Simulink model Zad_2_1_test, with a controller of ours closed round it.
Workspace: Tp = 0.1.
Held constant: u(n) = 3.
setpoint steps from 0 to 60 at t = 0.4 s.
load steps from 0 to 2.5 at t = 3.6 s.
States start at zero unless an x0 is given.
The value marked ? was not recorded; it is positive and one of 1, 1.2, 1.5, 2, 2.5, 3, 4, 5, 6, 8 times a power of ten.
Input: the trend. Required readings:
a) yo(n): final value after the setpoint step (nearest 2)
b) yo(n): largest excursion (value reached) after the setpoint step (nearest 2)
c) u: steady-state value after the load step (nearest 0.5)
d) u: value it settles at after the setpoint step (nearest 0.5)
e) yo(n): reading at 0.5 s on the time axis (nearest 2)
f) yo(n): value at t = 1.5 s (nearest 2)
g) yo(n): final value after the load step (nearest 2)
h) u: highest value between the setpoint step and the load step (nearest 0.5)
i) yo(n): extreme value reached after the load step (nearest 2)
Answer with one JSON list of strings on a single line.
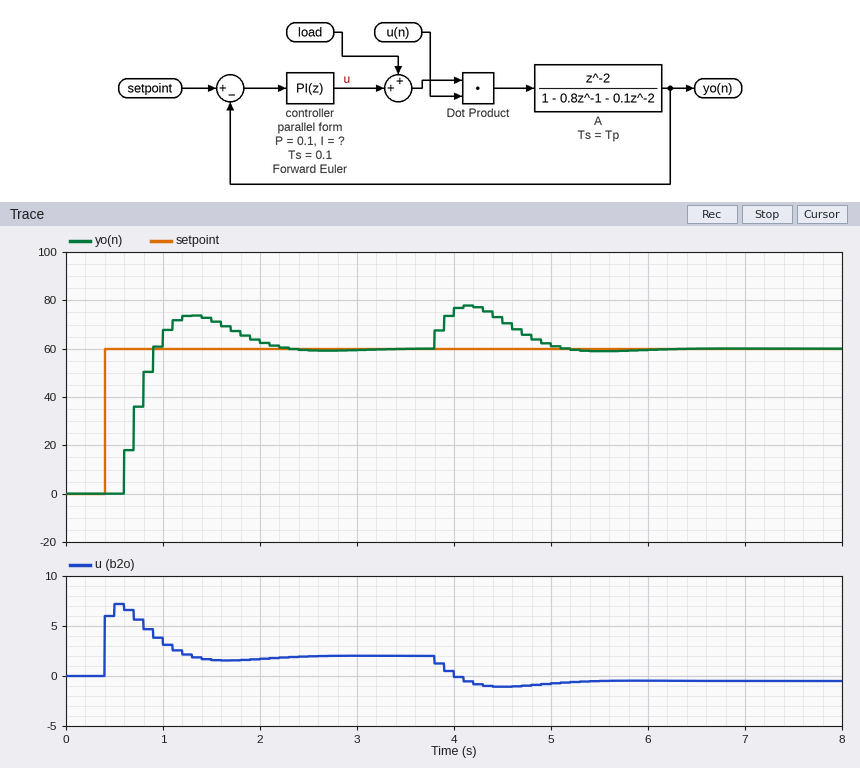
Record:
["60", "74", "-0.5", "2.0", "0", "72", "60", "7.0", "78"]
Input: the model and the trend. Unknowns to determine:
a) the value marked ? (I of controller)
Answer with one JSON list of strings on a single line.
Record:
["0.2"]
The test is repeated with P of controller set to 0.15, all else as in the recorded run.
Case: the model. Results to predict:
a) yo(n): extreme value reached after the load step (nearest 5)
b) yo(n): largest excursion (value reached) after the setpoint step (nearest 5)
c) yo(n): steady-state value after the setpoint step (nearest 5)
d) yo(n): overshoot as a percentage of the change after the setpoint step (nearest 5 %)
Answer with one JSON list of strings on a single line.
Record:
["75", "70", "60", "20 %"]
